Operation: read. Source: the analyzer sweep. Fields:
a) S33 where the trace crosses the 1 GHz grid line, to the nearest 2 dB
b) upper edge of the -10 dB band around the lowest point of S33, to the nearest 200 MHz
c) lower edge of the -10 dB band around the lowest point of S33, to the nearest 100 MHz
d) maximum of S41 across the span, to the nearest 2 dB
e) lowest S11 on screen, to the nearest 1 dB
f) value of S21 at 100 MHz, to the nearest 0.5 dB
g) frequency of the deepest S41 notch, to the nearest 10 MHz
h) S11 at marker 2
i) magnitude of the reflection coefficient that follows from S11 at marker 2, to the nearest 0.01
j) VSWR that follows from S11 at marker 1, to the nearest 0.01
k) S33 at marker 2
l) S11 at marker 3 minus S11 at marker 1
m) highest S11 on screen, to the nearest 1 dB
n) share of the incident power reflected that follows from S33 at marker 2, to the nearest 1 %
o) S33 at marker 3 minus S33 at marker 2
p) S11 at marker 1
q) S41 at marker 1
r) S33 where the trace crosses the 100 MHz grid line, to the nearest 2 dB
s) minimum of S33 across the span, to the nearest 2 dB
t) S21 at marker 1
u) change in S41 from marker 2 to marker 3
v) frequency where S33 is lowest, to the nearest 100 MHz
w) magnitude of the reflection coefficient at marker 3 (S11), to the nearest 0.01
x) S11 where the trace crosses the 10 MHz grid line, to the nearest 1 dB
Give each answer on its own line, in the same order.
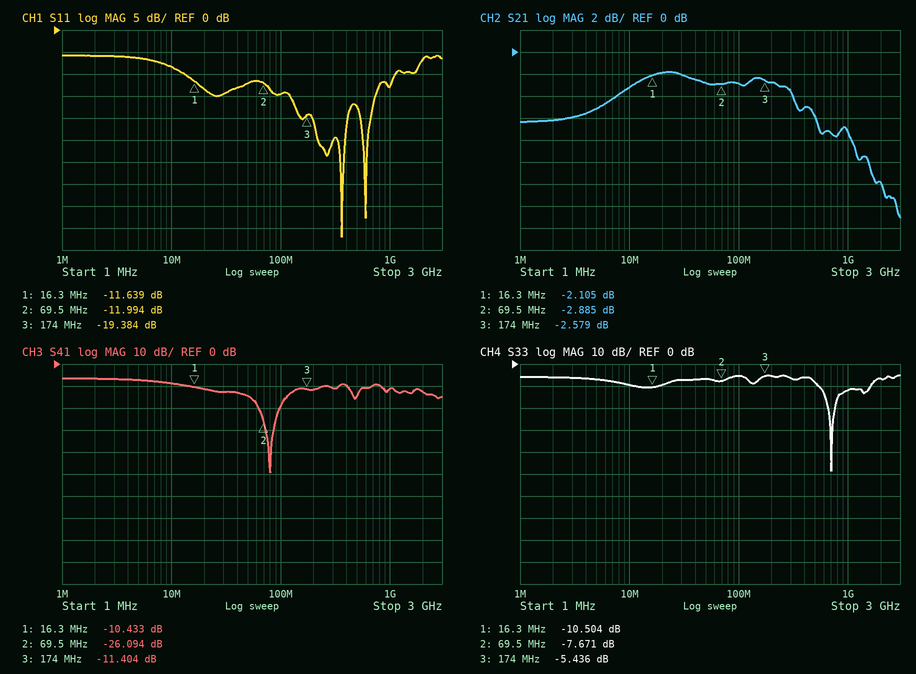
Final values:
-12 dB
1.6 GHz
500 MHz
-6 dB
-47 dB
-3.0 dB
80 MHz
-11.994 dB
0.25
1.71
-7.671 dB
-7.745 dB
-6 dB
17 %
2.235 dB
-11.639 dB
-10.433 dB
-6 dB
-48 dB
-2.105 dB
14.690 dB
700 MHz
0.11
-8 dB
